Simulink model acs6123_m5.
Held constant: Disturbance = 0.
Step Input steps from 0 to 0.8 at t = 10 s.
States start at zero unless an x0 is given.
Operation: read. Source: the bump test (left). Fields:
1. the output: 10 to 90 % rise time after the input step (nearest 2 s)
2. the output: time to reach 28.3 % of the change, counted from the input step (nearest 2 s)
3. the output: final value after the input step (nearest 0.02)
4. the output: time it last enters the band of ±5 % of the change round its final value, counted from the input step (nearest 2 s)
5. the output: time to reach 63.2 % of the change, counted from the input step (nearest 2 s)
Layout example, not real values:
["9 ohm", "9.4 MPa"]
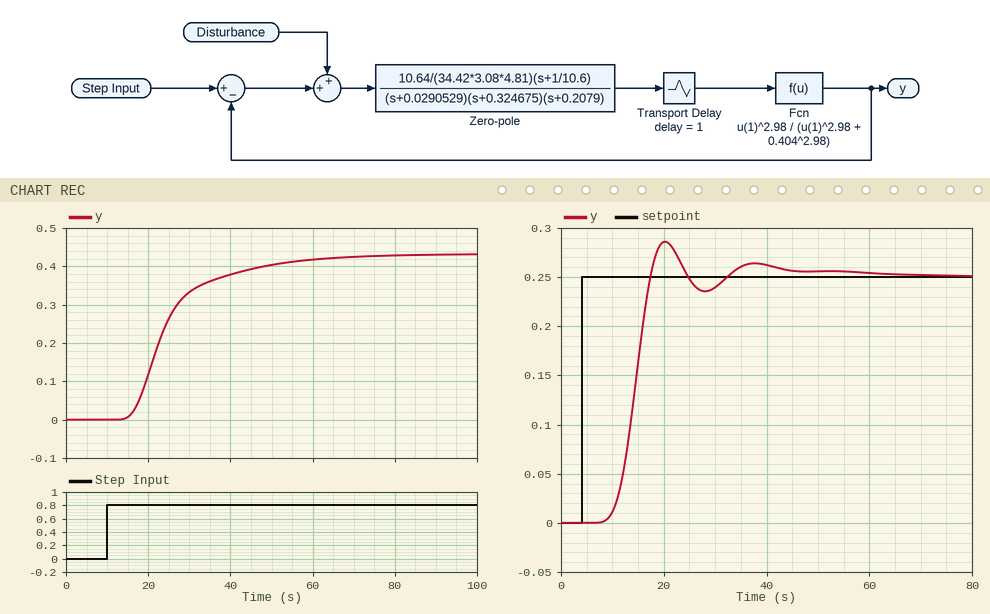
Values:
["26 s", "10 s", "0.44", "44 s", "16 s"]
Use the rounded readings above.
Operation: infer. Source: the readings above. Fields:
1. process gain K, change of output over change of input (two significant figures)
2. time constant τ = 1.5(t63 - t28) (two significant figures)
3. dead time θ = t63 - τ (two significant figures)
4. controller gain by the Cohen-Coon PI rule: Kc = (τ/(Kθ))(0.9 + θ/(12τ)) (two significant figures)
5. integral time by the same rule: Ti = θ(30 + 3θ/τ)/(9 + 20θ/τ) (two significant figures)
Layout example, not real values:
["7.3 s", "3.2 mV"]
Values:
["0.55", "9.0 s", "7.0 s", "2.3", "9.2 s"]
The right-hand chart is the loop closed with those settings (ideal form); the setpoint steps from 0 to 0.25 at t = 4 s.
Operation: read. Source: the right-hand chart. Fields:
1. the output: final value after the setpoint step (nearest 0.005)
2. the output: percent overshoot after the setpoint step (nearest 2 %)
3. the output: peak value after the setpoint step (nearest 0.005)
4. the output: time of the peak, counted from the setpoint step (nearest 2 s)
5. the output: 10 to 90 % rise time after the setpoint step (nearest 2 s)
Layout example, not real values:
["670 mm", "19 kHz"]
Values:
["0.250", "14 %", "0.285", "16 s", "6 s"]
